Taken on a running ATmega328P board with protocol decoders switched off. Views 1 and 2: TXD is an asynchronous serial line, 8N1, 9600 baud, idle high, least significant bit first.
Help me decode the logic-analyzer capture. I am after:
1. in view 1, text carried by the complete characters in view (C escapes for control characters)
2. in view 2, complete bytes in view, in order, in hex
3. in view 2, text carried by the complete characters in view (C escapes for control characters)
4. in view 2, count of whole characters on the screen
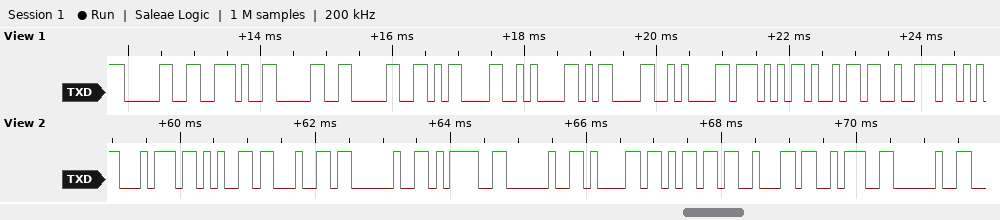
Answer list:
"0.00\r\n\r\nWir"
74 65 64 20 3D 20 61 6D 62 3A 20
"ted = amb: "
11
